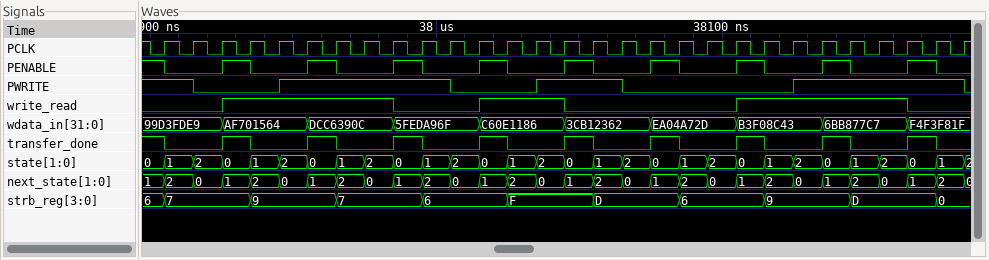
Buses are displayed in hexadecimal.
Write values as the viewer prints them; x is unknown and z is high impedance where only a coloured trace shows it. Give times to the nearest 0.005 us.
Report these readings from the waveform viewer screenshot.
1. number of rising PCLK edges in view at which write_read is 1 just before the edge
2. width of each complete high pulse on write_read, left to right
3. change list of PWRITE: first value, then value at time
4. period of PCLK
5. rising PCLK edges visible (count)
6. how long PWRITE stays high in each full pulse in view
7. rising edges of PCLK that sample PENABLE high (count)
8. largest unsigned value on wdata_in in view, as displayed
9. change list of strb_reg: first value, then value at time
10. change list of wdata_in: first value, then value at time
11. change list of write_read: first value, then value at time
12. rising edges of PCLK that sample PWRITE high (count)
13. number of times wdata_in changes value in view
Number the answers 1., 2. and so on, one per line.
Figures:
1. 15
2. 0.06 us, 0.03 us, 0.06 us
3. 1, 0 at 37.915 us, 1 at 37.945 us, 0 at 38.005 us, 1 at 38.035 us, 0 at 38.065 us, 1 at 38.125 us, 0 at 38.185 us
4. 0.01 us
5. 29
6. 0.06 us, 0.03 us, 0.06 us
7. 10
8. F4F3F81F
9. 6, 7 at 37.905 us, 9 at 37.935 us, 7 at 37.965 us, 6 at 37.995 us, F at 38.025 us, D at 38.055 us, 6 at 38.085 us, 9 at 38.115 us, D at 38.145 us, 0 at 38.175 us
10. 99D3FDE9, AF701564 at 37.925 us, DCC6390C at 37.955 us, 5FEDA96F at 37.985 us, C60E1186 at 38.015 us, 3CB12362 at 38.045 us, EA04A72D at 38.075 us, B3F08C43 at 38.105 us, 6BB877C7 at 38.135 us, F4F3F81F at 38.165 us
11. 0, 1 at 37.925 us, 0 at 37.985 us, 1 at 38.015 us, 0 at 38.045 us, 1 at 38.105 us, 0 at 38.165 us
12. 17
13. 9
